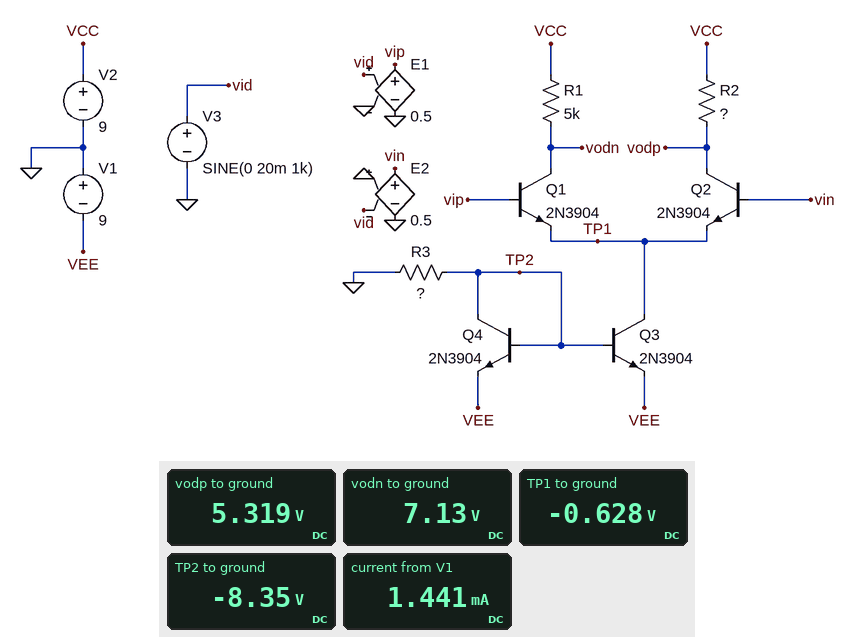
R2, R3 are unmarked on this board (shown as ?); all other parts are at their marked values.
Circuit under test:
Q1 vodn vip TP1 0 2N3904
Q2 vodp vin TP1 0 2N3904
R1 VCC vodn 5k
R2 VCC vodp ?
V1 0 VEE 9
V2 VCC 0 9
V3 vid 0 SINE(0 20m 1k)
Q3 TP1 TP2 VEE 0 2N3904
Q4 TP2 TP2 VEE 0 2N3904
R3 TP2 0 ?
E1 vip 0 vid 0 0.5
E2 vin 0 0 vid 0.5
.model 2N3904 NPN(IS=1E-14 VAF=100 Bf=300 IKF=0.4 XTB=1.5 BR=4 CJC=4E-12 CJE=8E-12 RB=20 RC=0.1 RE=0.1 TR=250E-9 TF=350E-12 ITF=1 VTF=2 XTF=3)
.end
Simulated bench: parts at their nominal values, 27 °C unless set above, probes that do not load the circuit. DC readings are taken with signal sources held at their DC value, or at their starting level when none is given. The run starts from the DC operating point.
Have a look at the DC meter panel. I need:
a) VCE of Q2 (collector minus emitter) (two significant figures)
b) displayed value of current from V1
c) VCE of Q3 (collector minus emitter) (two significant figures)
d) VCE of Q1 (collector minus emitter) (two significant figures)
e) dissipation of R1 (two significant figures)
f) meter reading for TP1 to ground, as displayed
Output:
5.9 V
1.441 mA
8.4 V
7.8 V
700 µW
-0.628 V
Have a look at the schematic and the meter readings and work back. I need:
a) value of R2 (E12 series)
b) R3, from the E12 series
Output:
10 kΩ
12 kΩ
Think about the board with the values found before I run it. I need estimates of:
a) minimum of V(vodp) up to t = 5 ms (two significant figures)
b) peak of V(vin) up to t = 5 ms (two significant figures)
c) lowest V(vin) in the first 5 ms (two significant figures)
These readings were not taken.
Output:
4.0 V
10 mV
-10 mV
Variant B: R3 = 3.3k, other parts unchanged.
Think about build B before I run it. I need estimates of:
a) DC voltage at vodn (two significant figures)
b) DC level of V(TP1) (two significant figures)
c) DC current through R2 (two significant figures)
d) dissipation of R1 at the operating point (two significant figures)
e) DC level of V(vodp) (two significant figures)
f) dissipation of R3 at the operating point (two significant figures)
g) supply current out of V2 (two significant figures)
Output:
910 mV
-670 mV
960 µA
13 mW
-630 mV
21 mW
2.6 mA
